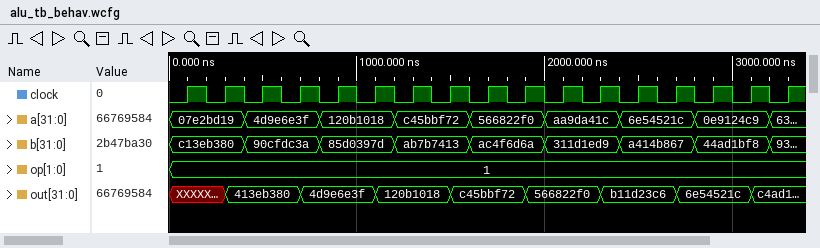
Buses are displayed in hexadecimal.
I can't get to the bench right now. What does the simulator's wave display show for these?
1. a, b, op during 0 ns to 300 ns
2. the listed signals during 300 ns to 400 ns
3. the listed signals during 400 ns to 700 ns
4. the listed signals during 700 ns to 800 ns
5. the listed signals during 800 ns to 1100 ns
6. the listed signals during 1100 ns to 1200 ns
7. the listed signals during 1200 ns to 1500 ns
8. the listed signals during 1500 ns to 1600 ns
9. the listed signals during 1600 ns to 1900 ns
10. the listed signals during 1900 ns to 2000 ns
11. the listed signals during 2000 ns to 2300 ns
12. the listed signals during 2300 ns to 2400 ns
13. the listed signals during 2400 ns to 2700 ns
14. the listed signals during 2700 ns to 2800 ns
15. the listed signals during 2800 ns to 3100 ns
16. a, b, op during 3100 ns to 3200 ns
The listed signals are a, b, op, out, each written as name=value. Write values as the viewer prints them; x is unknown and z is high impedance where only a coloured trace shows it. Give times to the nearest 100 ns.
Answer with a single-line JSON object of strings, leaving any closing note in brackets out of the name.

{"a, b, op during 0 ns to 300 ns": "a=07e2bd19, b=c13eb380, op=1", "the listed signals during 300 ns to 400 ns": "a=07e2bd19, b=c13eb380, op=1, out=413eb380", "the listed signals during 400 ns to 700 ns": "a=4d9e6e3f, b=90cfdc3a, op=1, out=413eb380", "the listed signals during 700 ns to 800 ns": "a=4d9e6e3f, b=90cfdc3a, op=1, out=4d9e6e3f", "the listed signals during 800 ns to 1100 ns": "a=120b1018, b=85d0397d, op=1, out=4d9e6e3f", "the listed signals during 1100 ns to 1200 ns": "a=120b1018, b=85d0397d, op=1, out=120b1018", "the listed signals during 1200 ns to 1500 ns": "a=c45bbf72, b=ab7b7413, op=1, out=120b1018", "the listed signals during 1500 ns to 1600 ns": "a=c45bbf72, b=ab7b7413, op=1, out=c45bbf72", "the listed signals during 1600 ns to 1900 ns": "a=566822f0, b=ac4f6d6a, op=1, out=c45bbf72", "the listed signals during 1900 ns to 2000 ns": "a=566822f0, b=ac4f6d6a, op=1, out=566822f0", "the listed signals during 2000 ns to 2300 ns": "a=aa9da41c, b=311d1ed9, op=1, out=566822f0", "the listed signals during 2300 ns to 2400 ns": "a=aa9da41c, b=311d1ed9, op=1, out=b11d23c6", "the listed signals during 2400 ns to 2700 ns": "a=6e54521c, b=a414b867, op=1, out=b11d23c6", "the listed signals during 2700 ns to 2800 ns": "a=6e54521c, b=a414b867, op=1, out=6e54521c", "the listed signals during 2800 ns to 3100 ns": "a=0e9124c9, b=44ad1bf8, op=1, out=6e54521c", "a, b, op during 3100 ns to 3200 ns": "a=0e9124c9, b=44ad1bf8, op=1"}
